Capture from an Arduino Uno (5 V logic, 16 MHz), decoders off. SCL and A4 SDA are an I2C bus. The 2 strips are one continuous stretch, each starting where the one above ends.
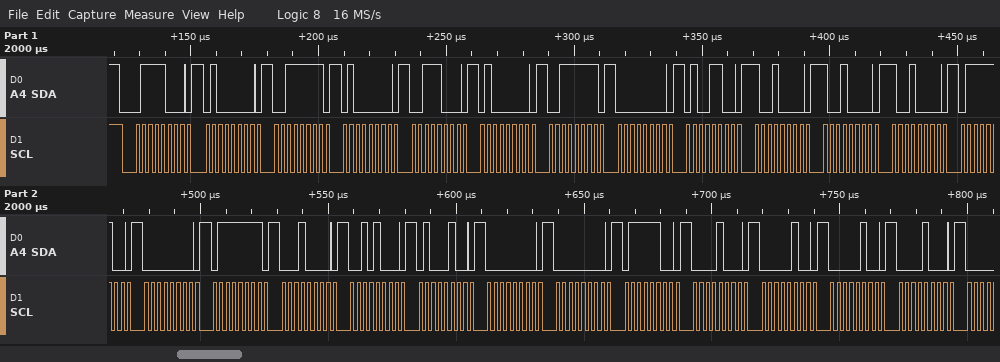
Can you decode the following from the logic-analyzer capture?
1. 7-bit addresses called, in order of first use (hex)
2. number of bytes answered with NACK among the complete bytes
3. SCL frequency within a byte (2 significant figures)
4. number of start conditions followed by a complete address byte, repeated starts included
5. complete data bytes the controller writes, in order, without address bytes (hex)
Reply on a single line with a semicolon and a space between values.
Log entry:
0x3C; 0; 400 kHz; 1; 40 3F 40 38 40 3F 00 4C 90 90 90 7C 00 7F 10 28 44 00 00 7C 08 04 04 08
